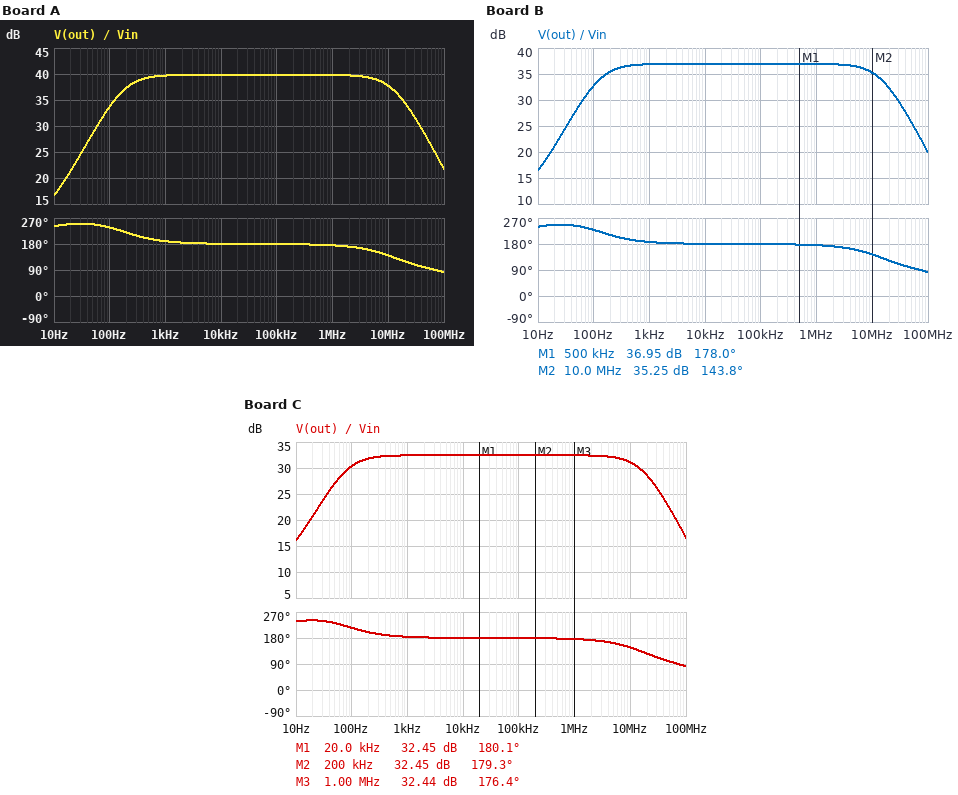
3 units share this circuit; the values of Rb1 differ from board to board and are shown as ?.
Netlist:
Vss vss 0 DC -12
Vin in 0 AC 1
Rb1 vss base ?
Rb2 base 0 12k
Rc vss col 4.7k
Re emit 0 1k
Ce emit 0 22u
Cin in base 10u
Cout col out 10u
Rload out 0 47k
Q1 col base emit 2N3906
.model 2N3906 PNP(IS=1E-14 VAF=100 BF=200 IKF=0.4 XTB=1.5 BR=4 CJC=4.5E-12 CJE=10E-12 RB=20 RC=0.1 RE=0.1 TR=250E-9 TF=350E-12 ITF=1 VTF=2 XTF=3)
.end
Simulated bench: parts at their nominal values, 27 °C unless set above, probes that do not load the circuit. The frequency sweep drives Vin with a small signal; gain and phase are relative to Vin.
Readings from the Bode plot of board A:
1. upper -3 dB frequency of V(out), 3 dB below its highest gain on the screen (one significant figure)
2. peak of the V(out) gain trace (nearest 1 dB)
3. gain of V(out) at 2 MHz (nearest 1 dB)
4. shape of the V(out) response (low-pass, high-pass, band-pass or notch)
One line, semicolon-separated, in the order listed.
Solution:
10 MHz; 40 dB; 40 dB; band-pass
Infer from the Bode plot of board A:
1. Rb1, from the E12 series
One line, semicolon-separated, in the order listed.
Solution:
100 kΩ
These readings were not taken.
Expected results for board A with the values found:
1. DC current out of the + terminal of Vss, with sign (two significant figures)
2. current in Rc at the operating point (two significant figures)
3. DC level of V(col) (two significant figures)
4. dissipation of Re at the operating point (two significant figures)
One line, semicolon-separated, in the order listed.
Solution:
-720 µA; 610 µA; -9.1 V; 380 µW
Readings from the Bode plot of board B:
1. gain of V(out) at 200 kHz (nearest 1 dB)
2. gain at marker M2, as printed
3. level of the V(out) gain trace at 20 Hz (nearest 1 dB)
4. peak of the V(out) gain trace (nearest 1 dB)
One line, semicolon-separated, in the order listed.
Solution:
37 dB; 35.25 dB; 21 dB; 37 dB
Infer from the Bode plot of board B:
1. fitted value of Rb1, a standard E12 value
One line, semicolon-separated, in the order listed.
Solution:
120 kΩ
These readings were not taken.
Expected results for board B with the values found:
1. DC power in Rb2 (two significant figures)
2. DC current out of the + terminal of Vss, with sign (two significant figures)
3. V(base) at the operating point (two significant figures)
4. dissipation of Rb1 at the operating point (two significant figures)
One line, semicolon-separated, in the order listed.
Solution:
95 µW; -530 µA; -1.1 V; 1.0 mW
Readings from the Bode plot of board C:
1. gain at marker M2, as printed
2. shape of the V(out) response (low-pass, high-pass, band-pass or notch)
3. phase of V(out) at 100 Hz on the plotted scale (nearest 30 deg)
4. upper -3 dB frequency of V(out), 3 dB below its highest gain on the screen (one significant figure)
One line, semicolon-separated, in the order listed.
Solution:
32.45 dB; band-pass; 210 deg; 20 MHz
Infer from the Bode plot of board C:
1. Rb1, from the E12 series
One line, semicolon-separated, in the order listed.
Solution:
150 kΩ
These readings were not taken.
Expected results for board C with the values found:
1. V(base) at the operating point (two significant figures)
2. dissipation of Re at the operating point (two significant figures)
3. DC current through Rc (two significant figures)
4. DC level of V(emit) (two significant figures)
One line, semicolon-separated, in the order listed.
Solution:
-880 mV; 67 µW; 260 µA; -260 mV
